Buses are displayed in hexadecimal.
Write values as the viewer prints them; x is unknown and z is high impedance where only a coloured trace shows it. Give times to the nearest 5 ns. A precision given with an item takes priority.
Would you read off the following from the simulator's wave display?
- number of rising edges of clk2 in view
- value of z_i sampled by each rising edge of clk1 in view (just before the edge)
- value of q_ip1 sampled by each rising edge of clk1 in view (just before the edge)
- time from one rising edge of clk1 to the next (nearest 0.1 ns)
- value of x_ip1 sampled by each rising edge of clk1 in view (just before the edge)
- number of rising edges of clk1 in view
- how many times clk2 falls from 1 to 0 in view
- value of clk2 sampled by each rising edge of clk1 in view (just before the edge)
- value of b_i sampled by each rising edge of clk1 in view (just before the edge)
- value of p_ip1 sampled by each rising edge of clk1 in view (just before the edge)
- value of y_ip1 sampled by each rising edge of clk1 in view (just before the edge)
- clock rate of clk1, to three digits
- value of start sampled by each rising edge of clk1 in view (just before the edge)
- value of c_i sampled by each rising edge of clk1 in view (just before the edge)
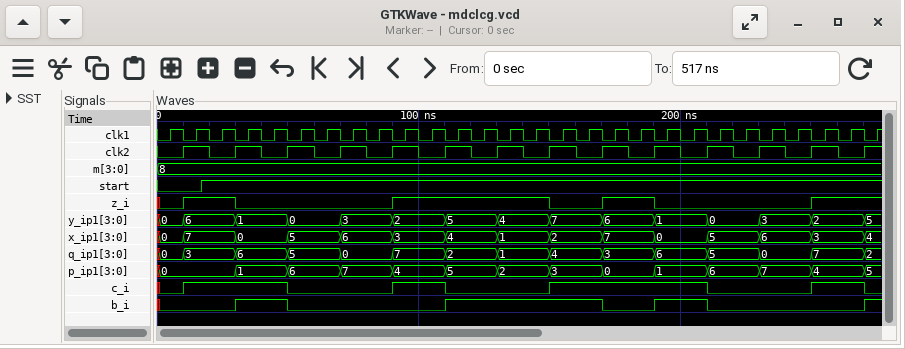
14
0 1 1 0 0 0 0 0 0 1 1 1 1 1 1 0 0 1 1 0 0 0 0 0 0 1 1 1
0, 3, 3, 6, 6, 5, 5, 0, 0, 7, 7, 2, 2, 1, 1, 4, 4, 3, 3, 6, 6, 5, 5, 0, 0, 7, 7, 2
10 ns
0, 7, 7, 0, 0, 5, 5, 6, 6, 3, 3, 4, 4, 1, 1, 2, 2, 7, 7, 0, 0, 5, 5, 6, 6, 3, 3, 4
28
13
0 1 0 1 0 1 0 1 0 1 0 1 0 1 0 1 0 1 0 1 0 1 0 1 0 1 0 1
0 0 0 1 1 0 0 0 0 0 0 1 1 1 1 1 1 0 0 1 1 0 0 0 0 0 0 1
0, 0, 0, 1, 1, 6, 6, 7, 7, 4, 4, 5, 5, 2, 2, 3, 3, 0, 0, 1, 1, 6, 6, 7, 7, 4, 4, 5
0, 6, 6, 1, 1, 0, 0, 3, 3, 2, 2, 5, 5, 4, 4, 7, 7, 6, 6, 1, 1, 0, 0, 3, 3, 2, 2, 5
100 MHz
0 0 1 1 1 1 1 1 1 1 1 1 1 1 1 1 1 1 1 1 1 1 1 1 1 1 1 1
0 1 1 1 1 0 0 0 0 1 1 0 0 0 0 1 1 1 1 1 1 0 0 0 0 1 1 0
